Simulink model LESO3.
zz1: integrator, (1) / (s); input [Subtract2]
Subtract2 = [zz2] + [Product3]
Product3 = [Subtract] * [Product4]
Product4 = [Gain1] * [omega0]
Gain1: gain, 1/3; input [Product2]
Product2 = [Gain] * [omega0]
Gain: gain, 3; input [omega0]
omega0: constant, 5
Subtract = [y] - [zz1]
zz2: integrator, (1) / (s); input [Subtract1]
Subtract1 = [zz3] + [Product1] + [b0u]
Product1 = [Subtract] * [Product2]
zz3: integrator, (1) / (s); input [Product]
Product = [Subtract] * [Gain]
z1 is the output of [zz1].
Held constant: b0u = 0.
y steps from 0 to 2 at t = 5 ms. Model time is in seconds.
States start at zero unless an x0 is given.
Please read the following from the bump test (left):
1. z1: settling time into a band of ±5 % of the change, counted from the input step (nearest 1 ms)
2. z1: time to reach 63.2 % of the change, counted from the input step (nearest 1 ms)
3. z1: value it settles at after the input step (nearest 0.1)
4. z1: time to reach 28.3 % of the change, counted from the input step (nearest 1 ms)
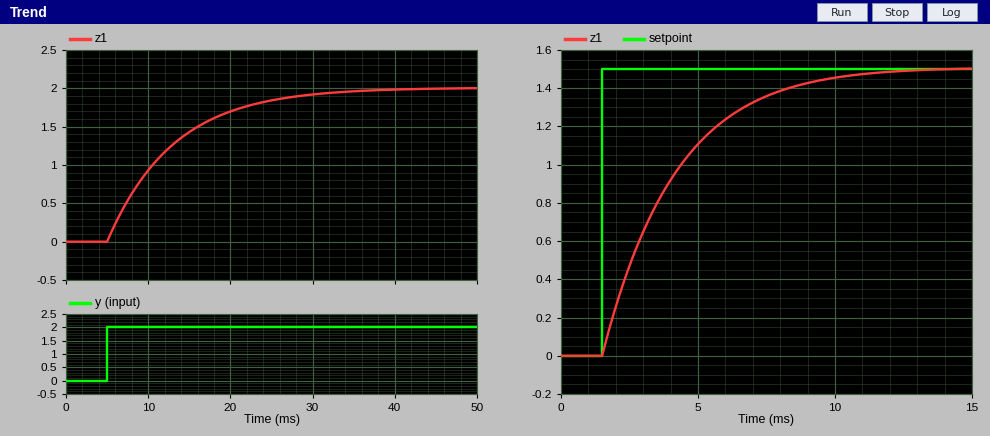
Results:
24 ms
8 ms
2.0
3 ms
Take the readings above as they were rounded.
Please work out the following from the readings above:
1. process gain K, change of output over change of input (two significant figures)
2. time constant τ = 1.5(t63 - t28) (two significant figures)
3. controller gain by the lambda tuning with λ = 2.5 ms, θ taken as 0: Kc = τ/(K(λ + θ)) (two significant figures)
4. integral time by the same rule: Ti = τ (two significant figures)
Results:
1.0
7.5 ms
3.0
7.5 ms
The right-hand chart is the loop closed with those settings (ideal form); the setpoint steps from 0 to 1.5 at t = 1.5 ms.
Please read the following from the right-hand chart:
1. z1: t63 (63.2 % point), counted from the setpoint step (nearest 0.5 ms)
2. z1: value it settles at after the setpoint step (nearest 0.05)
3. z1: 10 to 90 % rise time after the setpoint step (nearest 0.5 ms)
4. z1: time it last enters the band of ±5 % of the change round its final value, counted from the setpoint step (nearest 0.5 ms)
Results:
2.5 ms
1.50
5.5 ms
7.5 ms
